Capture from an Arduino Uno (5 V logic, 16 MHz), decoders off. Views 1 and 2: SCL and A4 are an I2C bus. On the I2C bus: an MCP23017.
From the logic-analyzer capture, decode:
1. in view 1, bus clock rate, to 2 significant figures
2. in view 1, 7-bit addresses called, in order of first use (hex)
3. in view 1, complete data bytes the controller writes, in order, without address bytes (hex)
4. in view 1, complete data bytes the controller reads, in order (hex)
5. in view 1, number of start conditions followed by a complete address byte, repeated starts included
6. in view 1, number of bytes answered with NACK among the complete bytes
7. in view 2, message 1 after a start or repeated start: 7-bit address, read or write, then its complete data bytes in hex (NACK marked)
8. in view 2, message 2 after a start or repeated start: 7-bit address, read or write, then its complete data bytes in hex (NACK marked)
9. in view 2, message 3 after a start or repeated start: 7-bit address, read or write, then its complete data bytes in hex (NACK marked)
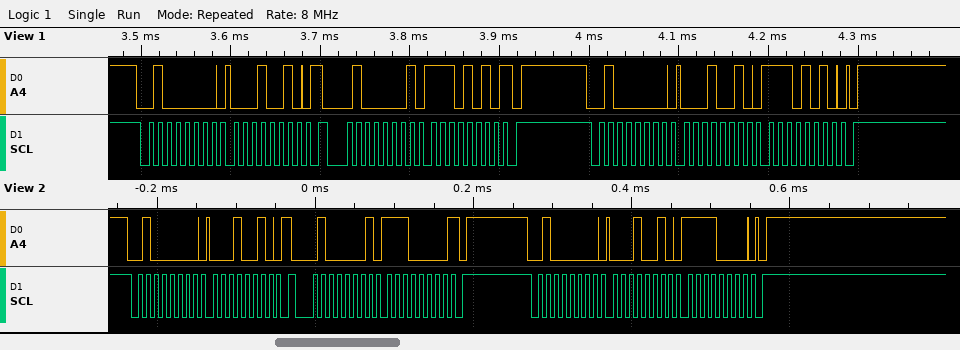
100 kHz
0x20
12 12 EA
EA
3
1
0x20 write: 12
0x20 read: E0 NACK
0x20 write: 12 F0
